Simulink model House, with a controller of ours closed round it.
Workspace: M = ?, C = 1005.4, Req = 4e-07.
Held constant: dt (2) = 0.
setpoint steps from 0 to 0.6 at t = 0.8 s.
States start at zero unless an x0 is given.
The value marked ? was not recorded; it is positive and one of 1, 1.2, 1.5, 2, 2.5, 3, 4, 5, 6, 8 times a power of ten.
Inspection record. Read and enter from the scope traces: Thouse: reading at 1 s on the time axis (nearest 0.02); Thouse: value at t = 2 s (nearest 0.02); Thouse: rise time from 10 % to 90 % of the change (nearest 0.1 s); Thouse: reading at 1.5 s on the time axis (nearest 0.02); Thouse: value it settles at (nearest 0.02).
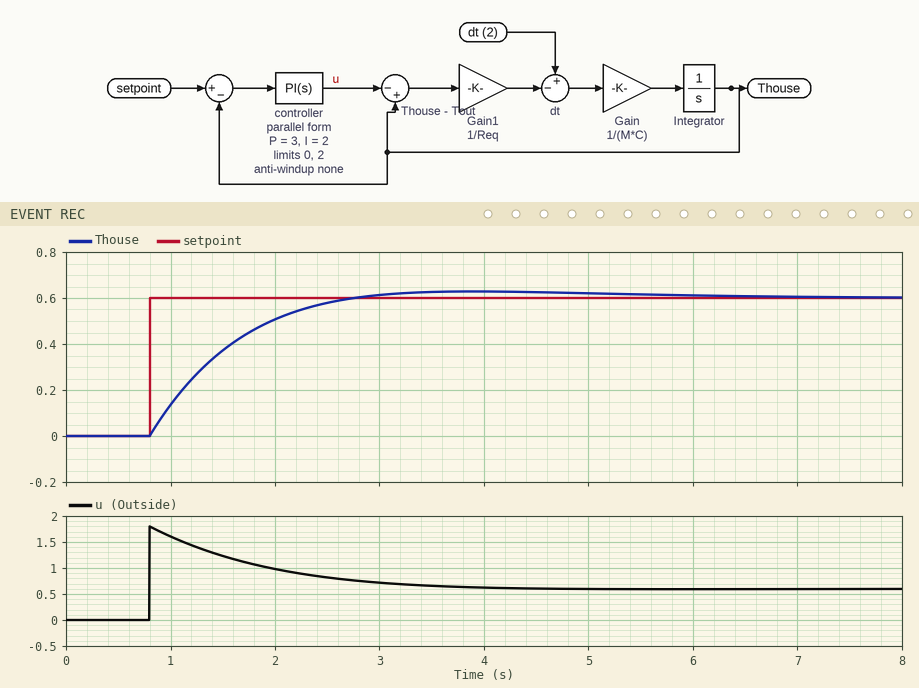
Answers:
0.14
0.50
1.3 s
0.38
0.60
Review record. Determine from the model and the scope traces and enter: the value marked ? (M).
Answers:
6000
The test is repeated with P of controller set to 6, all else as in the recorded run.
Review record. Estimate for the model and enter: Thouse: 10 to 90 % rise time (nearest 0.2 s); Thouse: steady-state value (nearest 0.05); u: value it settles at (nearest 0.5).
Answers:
1.0 s
0.60
0.5
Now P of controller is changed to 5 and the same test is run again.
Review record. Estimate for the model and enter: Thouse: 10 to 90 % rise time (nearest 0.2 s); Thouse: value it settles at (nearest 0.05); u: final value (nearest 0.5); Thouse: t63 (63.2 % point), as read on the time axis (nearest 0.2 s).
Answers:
1.0 s
0.60
0.5
1.4 s
